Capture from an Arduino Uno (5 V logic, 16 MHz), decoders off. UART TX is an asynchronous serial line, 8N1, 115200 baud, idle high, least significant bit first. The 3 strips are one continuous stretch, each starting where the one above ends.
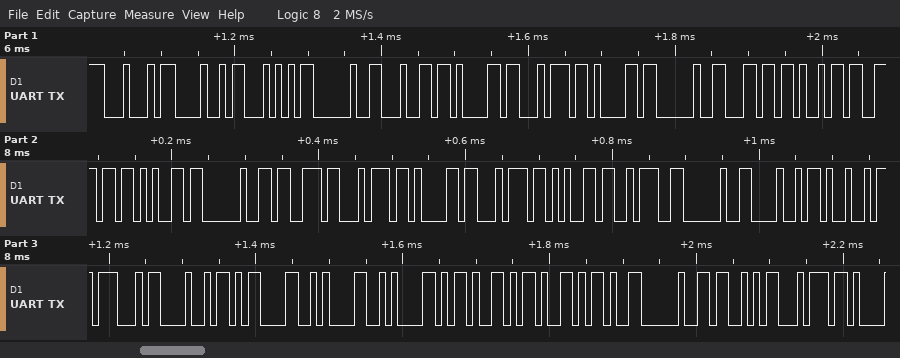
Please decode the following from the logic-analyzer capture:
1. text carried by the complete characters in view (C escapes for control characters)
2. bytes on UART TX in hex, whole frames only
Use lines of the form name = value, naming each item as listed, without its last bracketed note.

text carried by the complete characters in view = "DHT data line state: HIGH\r\n\n--- St"
bytes on UART TX in hex, whole frames only = 0x44 0x48 0x54 0x20 0x64 0x61 0x74 0x61 0x20 0x6C 0x69 0x6E 0x65 0x20 0x73 0x74 0x61 0x74 0x65 0x3A 0x20 0x48 0x49 0x47 0x48 0x0D 0x0A 0x0A 0x2D 0x2D 0x2D 0x20 0x53 0x74
